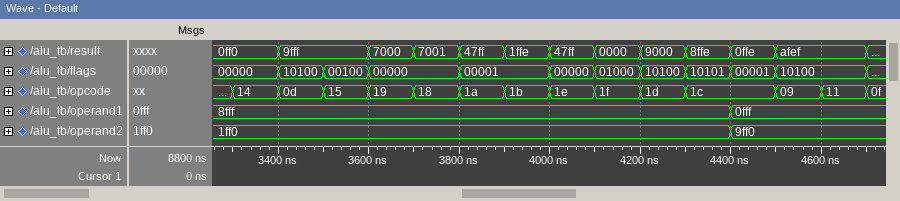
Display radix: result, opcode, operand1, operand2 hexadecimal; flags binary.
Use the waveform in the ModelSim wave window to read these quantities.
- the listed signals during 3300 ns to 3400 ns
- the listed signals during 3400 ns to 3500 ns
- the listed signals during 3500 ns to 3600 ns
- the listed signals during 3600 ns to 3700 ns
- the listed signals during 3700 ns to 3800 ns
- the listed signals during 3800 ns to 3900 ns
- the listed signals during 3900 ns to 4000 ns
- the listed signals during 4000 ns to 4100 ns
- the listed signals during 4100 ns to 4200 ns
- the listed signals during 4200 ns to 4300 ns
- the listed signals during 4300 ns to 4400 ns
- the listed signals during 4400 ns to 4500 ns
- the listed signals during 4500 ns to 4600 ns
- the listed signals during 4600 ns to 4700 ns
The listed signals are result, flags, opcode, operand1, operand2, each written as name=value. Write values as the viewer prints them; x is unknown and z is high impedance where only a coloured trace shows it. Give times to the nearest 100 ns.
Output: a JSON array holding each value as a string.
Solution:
["result=0ff0, flags=00000, opcode=14, operand1=8fff, operand2=1ff0", "result=9fff, flags=10100, opcode=0d, operand1=8fff, operand2=1ff0", "result=9fff, flags=00100, opcode=15, operand1=8fff, operand2=1ff0", "result=7000, flags=00000, opcode=19, operand1=8fff, operand2=1ff0", "result=7001, flags=00000, opcode=18, operand1=8fff, operand2=1ff0", "result=47ff, flags=00001, opcode=1a, operand1=8fff, operand2=1ff0", "result=1ffe, flags=00001, opcode=1b, operand1=8fff, operand2=1ff0", "result=47ff, flags=00000, opcode=1e, operand1=8fff, operand2=1ff0", "result=0000, flags=01000, opcode=1f, operand1=8fff, operand2=1ff0", "result=9000, flags=10100, opcode=1d, operand1=8fff, operand2=1ff0", "result=8ffe, flags=10101, opcode=1c, operand1=8fff, operand2=1ff0", "result=0ffe, flags=00001, opcode=1c, operand1=0fff, operand2=9ff0", "result=afef, flags=10100, opcode=09, operand1=0fff, operand2=9ff0", "result=afef, flags=10100, opcode=11, operand1=0fff, operand2=9ff0"]
